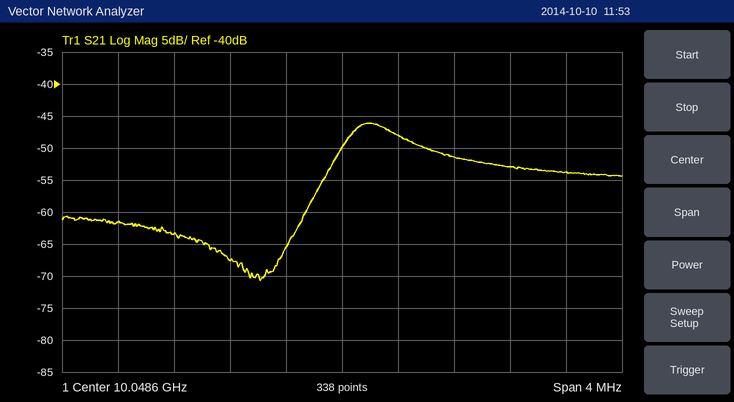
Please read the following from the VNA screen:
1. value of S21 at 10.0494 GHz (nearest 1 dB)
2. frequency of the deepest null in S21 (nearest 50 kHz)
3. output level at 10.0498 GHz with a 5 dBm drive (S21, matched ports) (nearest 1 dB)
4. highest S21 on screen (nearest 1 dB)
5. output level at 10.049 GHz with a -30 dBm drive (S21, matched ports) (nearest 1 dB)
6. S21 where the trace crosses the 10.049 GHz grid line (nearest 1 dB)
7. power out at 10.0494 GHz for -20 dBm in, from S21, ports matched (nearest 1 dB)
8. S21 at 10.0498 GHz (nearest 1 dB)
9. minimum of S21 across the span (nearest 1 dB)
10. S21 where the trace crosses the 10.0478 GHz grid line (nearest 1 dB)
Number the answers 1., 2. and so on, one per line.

1. -51 dB
2. 10.04800 GHz
3. -48 dBm
4. -46 dB
5. -78 dBm
6. -48 dB
7. -71 dBm
8. -53 dB
9. -71 dB
10. -68 dB
